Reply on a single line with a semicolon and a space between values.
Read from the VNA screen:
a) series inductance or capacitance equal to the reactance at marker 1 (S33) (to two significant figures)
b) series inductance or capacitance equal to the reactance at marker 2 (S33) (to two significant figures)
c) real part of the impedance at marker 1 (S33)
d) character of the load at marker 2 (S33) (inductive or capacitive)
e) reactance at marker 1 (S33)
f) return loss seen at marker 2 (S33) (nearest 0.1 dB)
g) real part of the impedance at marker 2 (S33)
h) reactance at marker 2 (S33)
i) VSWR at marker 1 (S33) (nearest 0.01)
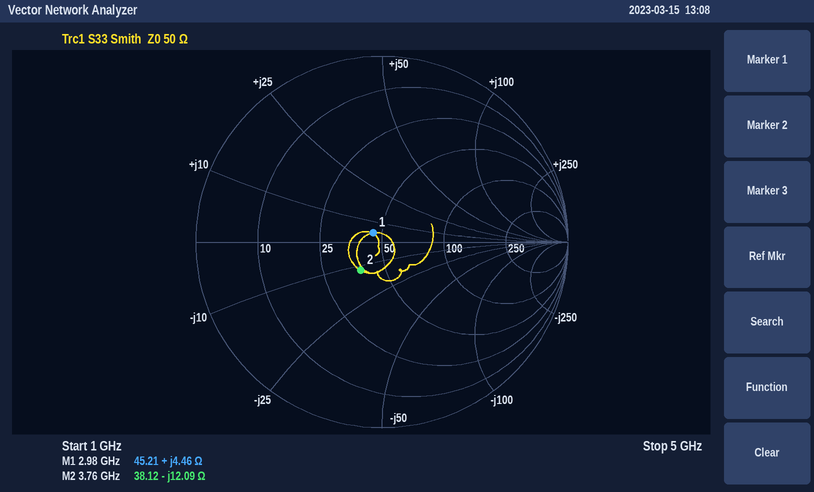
240 pH; 3.5 pF; 45.21 Ω; capacitive; +4.46 Ω; 14.4 dB; 38.12 Ω; -12.09 Ω; 1.15
